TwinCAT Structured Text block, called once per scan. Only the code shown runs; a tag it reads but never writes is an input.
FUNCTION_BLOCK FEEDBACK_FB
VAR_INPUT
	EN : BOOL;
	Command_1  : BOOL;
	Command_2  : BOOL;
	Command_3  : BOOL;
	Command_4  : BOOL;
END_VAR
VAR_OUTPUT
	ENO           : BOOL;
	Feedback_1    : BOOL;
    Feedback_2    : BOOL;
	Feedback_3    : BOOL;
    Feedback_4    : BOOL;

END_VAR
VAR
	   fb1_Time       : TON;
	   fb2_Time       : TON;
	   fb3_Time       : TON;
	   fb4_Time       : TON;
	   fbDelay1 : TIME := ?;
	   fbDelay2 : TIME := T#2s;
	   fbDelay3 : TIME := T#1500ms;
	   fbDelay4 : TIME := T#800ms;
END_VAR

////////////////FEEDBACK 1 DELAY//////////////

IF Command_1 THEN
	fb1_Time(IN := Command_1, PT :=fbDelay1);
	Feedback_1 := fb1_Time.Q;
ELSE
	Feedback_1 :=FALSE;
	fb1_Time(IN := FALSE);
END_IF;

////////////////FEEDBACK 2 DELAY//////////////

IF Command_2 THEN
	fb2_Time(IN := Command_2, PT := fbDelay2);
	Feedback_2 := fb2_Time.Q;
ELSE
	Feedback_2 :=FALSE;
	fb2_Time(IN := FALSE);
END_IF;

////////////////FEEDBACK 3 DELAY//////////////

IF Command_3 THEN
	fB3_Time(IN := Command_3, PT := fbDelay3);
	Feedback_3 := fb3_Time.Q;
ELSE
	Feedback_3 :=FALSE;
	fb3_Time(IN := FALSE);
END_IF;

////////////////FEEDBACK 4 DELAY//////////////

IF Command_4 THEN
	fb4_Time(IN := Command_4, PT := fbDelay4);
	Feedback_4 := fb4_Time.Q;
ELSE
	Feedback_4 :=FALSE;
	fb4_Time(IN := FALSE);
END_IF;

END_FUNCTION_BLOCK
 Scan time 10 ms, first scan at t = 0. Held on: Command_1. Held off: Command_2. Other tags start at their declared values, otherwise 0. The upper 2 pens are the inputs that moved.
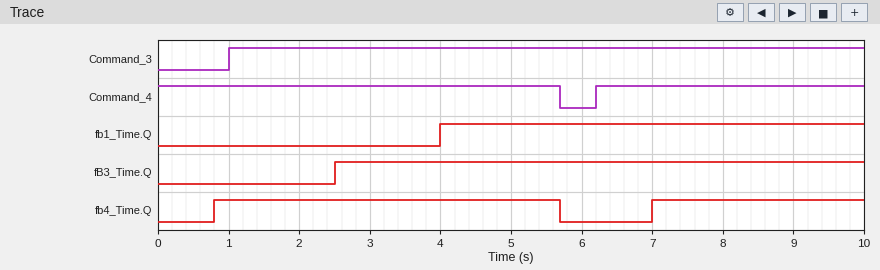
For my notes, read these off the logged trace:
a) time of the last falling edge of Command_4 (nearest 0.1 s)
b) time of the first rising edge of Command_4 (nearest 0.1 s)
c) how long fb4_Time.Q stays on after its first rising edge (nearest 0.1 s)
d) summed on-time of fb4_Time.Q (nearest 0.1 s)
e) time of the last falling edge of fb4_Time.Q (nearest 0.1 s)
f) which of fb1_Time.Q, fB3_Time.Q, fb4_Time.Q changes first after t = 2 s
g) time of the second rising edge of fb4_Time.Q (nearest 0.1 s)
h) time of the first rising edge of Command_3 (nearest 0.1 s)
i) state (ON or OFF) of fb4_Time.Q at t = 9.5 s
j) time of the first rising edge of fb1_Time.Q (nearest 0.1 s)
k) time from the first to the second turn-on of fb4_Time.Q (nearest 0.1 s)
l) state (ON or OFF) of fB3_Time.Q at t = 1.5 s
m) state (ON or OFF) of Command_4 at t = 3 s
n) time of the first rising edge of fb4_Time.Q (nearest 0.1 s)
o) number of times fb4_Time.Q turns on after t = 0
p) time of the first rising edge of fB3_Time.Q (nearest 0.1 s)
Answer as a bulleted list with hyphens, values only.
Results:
- 5.7 s
- 6.2 s
- 4.9 s
- 7.9 s
- 5.7 s
- fB3_Time.Q
- 7.0 s
- 1.0 s
- ON
- 4.0 s
- 6.2 s
- OFF
- ON
- 0.8 s
- 2
- 2.5 s
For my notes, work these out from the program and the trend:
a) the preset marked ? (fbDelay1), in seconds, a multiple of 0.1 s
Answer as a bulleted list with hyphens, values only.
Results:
- 4.0 s
